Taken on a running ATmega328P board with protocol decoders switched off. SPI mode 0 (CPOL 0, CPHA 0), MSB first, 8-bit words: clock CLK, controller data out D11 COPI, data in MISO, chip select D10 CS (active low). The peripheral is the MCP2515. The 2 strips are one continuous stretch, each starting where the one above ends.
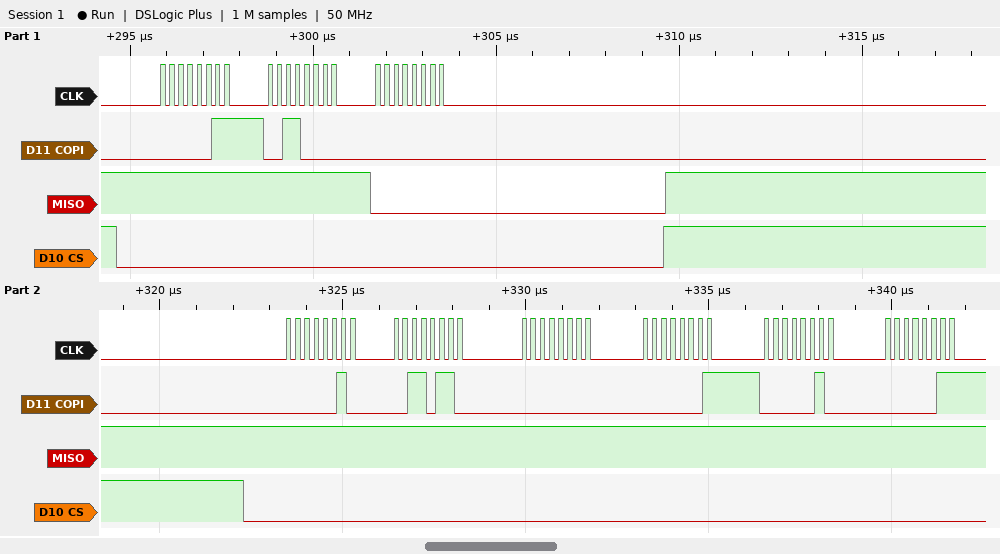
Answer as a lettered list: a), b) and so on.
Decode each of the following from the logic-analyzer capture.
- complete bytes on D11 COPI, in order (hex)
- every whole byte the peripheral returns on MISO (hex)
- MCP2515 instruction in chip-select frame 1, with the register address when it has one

a) 03 30 00 02 36 00 01 02 03
b) FF FF 00 FF FF FF FF FF FF
c) READ 0x30
